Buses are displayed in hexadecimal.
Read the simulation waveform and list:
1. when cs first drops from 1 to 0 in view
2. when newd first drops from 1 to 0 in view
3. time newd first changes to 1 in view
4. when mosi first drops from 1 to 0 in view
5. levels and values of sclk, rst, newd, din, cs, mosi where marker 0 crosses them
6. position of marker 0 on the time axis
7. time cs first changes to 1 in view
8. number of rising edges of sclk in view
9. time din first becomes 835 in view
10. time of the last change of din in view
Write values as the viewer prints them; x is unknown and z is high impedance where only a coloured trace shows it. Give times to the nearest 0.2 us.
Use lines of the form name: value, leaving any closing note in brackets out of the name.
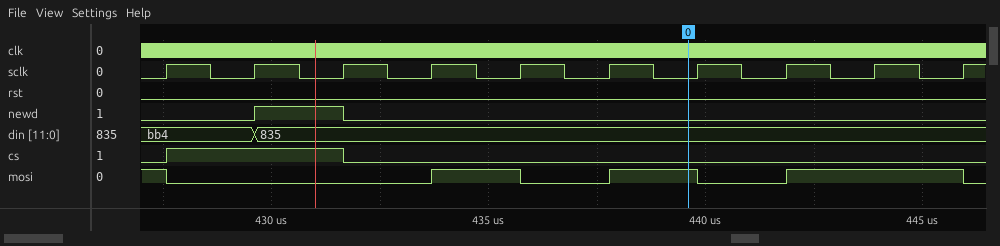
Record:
when cs first drops from 1 to 0 in view: 431.6 us
when newd first drops from 1 to 0 in view: 431.6 us
time newd first changes to 1 in view: 429.6 us
when mosi first drops from 1 to 0 in view: 427.6 us
levels and values of sclk, rst, newd, din, cs, mosi where marker 0 crosses them: sclk=0, rst=0, newd=0, din=835, cs=0, mosi=1
position of marker 0 on the time axis: 439.6 us
time cs first changes to 1 in view: 427.6 us
number of rising edges of sclk in view: 10
time din first becomes 835 in view: 429.6 us
time of the last change of din in view: 429.6 us
